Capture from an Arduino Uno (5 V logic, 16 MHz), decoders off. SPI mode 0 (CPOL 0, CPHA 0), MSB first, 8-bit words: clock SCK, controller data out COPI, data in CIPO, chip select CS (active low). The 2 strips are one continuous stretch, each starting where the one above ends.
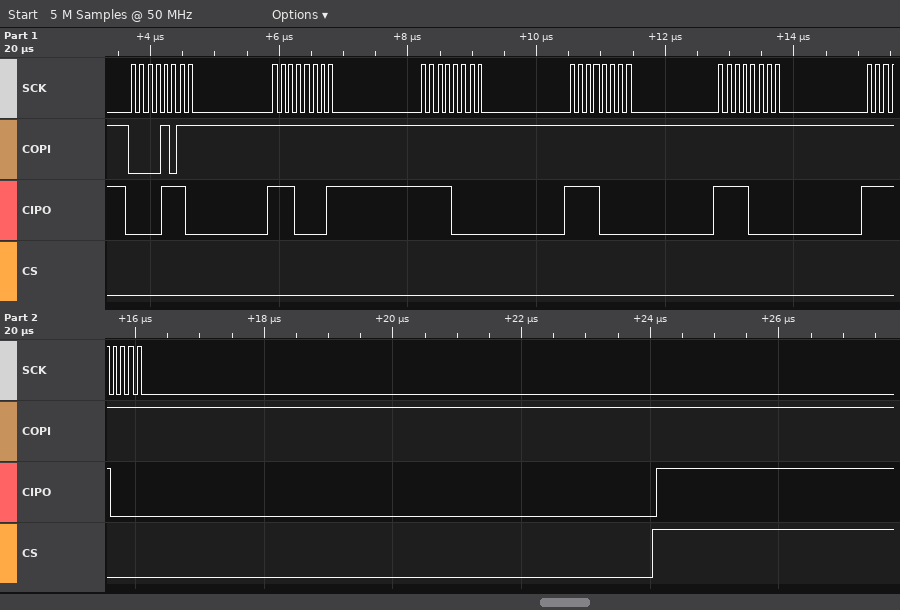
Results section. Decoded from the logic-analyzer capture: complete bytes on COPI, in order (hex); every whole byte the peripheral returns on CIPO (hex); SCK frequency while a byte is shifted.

0B FF FF FF FF FF
0E E1 F0 F0 F0 F0
8 MHz
